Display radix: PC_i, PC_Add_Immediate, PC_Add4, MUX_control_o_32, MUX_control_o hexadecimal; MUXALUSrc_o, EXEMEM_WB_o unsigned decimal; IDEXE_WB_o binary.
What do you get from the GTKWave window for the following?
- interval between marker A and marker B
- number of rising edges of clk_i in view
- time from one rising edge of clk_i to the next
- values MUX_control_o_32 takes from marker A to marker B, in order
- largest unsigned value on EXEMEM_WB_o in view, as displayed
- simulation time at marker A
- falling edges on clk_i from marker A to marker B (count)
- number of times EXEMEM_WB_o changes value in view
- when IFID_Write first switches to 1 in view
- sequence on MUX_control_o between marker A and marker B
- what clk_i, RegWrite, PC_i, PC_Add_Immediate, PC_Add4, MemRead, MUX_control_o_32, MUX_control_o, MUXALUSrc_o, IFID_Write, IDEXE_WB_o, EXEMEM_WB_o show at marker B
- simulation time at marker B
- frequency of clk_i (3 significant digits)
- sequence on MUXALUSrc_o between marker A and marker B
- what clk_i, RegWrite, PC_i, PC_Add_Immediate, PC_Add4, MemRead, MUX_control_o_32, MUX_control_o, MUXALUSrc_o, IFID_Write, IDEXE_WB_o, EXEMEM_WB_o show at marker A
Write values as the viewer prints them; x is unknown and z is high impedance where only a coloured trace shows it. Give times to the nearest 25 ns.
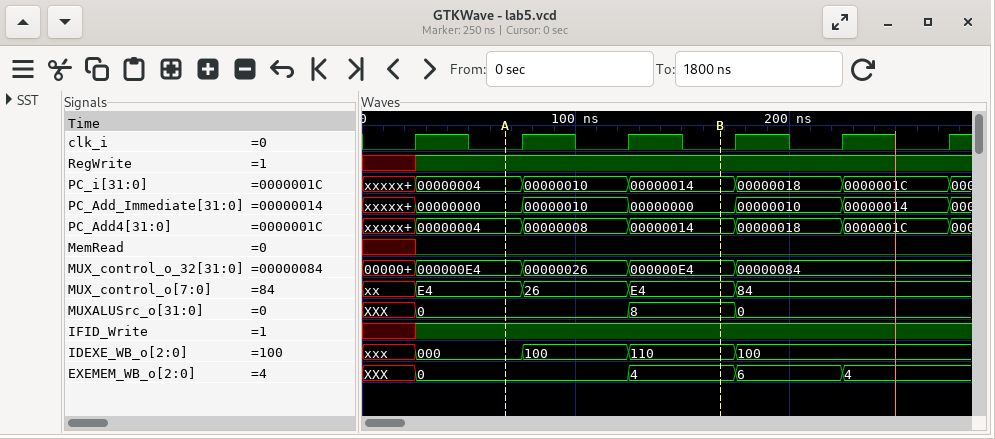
100 ns
6
50 ns
000000E4, 00000026, 000000E4
6
75 ns
2
4
25 ns
E4, 26, E4
clk_i=0, RegWrite=1, PC_i=00000014, PC_Add_Immediate=00000000, PC_Add4=00000014, MemRead=0, MUX_control_o_32=000000E4, MUX_control_o=E4, MUXALUSrc_o=8, IFID_Write=1, IDEXE_WB_o=110, EXEMEM_WB_o=4
175 ns
20.0 MHz
0, 8
clk_i=0, RegWrite=1, PC_i=00000004, PC_Add_Immediate=00000000, PC_Add4=00000004, MemRead=0, MUX_control_o_32=000000E4, MUX_control_o=E4, MUXALUSrc_o=0, IFID_Write=1, IDEXE_WB_o=000, EXEMEM_WB_o=0
